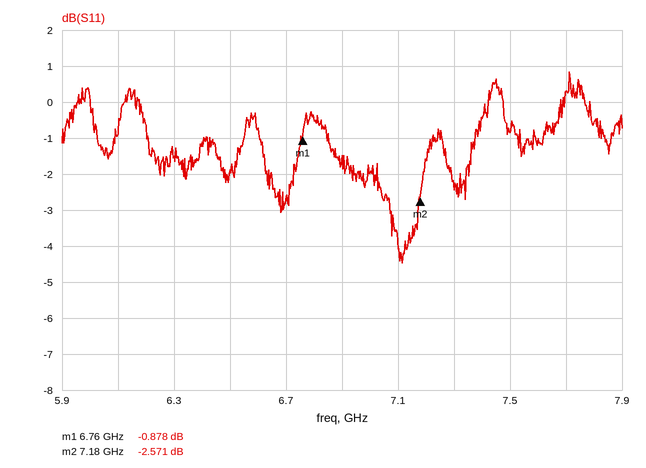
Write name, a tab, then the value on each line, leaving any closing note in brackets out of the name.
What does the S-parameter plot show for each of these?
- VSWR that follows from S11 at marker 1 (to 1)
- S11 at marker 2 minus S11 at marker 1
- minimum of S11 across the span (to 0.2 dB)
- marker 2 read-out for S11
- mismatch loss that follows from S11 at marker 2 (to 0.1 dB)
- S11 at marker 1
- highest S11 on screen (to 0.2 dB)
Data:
VSWR that follows from S11 at marker 1	20
S11 at marker 2 minus S11 at marker 1	-1.693 dB
minimum of S11 across the span	-4.4 dB
marker 2 read-out for S11	-2.571 dB
mismatch loss that follows from S11 at marker 2	3.5 dB
S11 at marker 1	-0.878 dB
highest S11 on screen	0.8 dB
